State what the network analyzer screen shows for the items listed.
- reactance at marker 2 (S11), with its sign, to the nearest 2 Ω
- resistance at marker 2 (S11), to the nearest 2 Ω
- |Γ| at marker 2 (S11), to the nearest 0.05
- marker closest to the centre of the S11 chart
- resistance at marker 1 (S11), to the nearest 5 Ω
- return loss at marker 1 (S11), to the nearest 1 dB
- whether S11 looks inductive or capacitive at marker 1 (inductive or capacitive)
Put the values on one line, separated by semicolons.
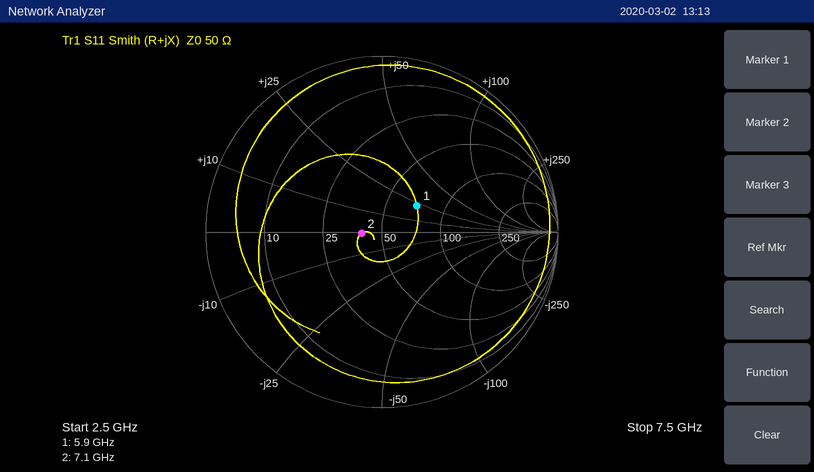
0 Ω; 40 Ω; 0.10; marker 2; 70 Ω; 12 dB; inductive
